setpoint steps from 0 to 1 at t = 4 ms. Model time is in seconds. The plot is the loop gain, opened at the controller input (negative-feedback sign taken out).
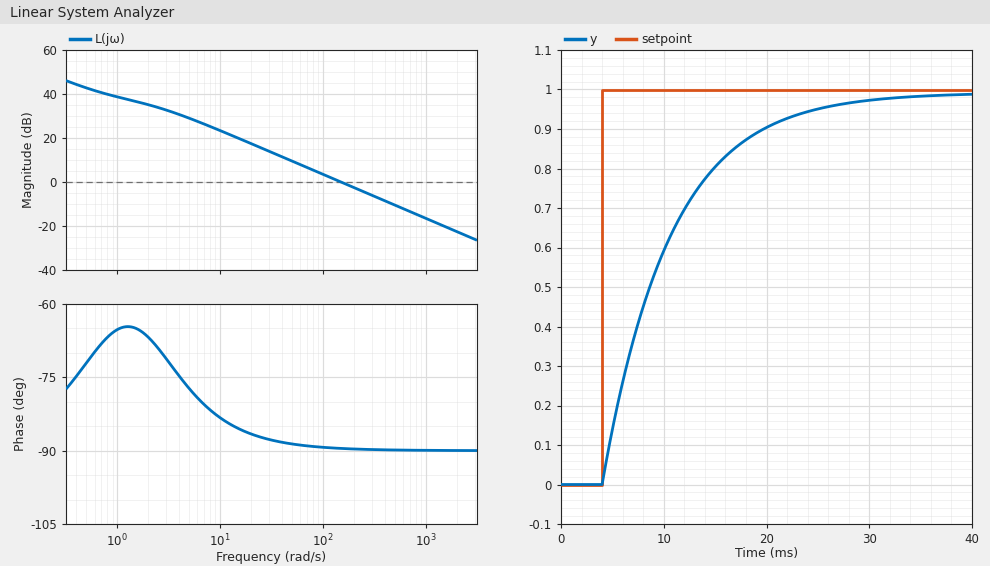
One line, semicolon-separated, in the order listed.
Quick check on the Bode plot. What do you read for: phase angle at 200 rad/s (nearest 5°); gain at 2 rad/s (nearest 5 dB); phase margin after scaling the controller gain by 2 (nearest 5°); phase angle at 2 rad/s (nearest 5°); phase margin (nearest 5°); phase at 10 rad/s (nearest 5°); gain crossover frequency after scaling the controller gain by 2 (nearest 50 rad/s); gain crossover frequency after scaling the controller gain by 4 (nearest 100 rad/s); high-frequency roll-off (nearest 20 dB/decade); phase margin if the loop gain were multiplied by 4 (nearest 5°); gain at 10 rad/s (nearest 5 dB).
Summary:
-90°; 35 dB; 90°; -65°; 90°; -85°; 300 rad/s; 600 rad/s; -20 dB/decade; 90°; 25 dB
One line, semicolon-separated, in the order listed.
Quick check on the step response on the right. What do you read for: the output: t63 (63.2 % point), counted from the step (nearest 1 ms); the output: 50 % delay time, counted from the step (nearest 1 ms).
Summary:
7 ms; 5 ms
